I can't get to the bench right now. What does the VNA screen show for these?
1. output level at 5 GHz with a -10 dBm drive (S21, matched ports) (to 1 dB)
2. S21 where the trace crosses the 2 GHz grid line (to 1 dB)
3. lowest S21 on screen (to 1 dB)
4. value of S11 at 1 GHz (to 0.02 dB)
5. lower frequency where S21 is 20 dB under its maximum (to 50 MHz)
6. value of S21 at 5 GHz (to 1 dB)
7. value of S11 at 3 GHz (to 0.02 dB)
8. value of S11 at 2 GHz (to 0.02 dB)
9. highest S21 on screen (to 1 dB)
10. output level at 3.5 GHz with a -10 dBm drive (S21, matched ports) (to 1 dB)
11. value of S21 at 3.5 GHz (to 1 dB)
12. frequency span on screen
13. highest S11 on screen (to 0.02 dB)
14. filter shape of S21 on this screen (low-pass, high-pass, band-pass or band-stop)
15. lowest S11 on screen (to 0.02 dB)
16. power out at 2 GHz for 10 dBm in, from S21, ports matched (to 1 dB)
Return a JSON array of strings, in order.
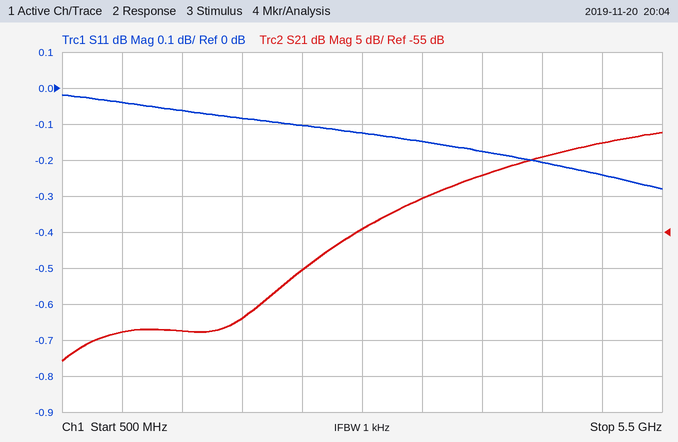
["-53 dBm", "-67 dB", "-73 dB", "-0.04 dB", "2.45 GHz", "-43 dB", "-0.12 dB", "-0.08 dB", "-41 dB", "-60 dBm", "-50 dB", "5 GHz", "-0.02 dB", "high-pass", "-0.28 dB", "-57 dBm"]
